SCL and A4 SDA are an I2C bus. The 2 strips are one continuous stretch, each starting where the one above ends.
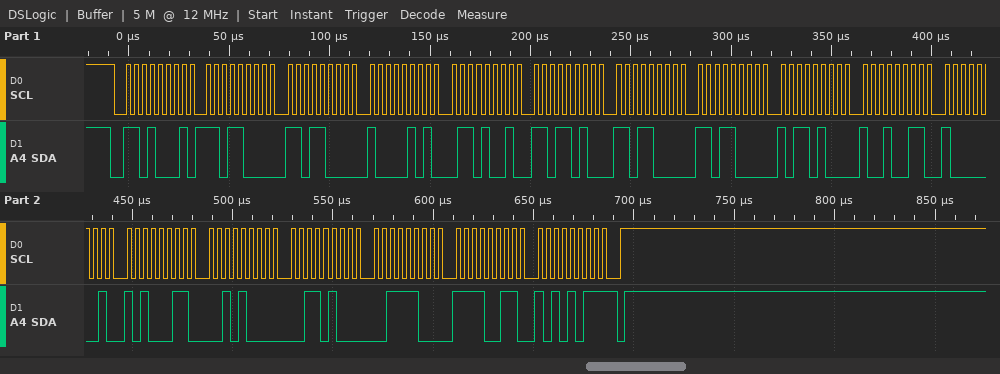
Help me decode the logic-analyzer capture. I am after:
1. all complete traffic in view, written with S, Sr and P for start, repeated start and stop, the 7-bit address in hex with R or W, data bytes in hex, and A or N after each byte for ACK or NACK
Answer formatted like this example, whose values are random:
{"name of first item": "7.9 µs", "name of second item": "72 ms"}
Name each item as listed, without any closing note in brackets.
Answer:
{"all complete traffic in view, written with S, Sr and P for start, repeated start and stop, the 7-bit address in hex with R or W, data bytes in hex, and A or N after each byte for ACK or NACK": "S 68R A D8 A D8 A 85 A 69 A DA A D8 A D8 A B4 A 93 A 81 A A3 A 28 A 34 A 3C A F3 A AB N P"}
